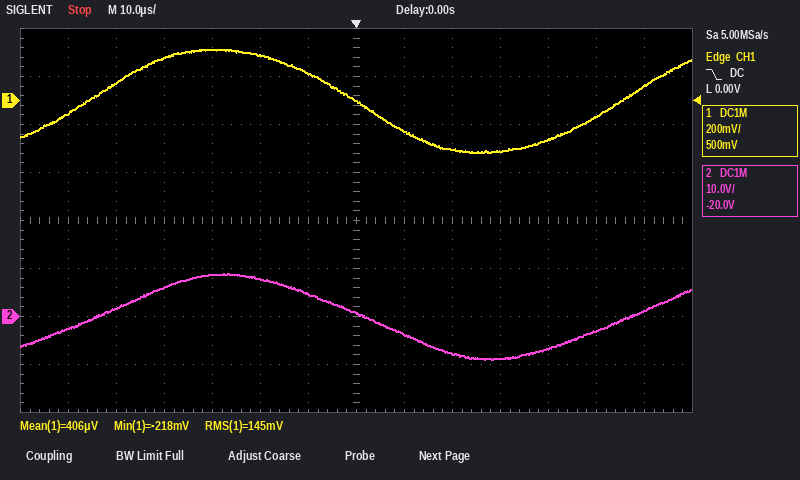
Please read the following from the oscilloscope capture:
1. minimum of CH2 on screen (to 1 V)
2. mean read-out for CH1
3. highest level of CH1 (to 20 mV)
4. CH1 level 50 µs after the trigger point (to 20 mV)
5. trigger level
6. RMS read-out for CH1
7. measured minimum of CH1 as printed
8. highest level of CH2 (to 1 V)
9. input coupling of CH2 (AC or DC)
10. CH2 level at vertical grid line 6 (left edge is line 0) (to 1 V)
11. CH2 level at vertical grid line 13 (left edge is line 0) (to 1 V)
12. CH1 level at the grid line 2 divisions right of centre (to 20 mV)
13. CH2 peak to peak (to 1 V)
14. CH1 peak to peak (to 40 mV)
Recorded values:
-9 V
406 µV
220 mV
-60 mV
0.00 V
145 mV
-218 mV
9 V
DC
5 V
1 V
-200 mV
18 V
440 mV
